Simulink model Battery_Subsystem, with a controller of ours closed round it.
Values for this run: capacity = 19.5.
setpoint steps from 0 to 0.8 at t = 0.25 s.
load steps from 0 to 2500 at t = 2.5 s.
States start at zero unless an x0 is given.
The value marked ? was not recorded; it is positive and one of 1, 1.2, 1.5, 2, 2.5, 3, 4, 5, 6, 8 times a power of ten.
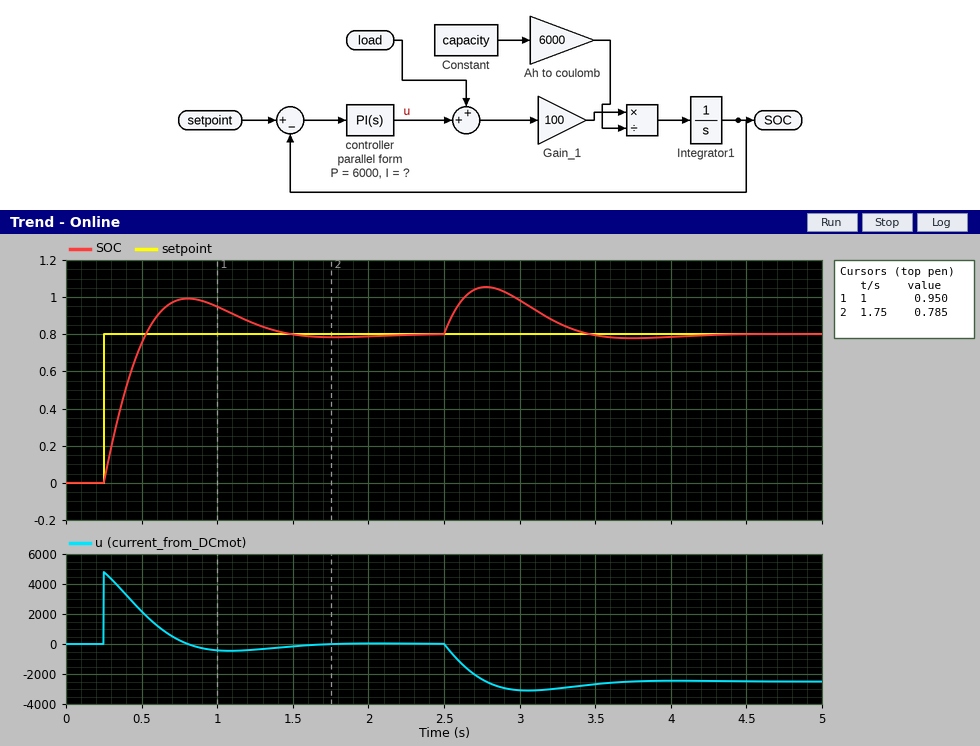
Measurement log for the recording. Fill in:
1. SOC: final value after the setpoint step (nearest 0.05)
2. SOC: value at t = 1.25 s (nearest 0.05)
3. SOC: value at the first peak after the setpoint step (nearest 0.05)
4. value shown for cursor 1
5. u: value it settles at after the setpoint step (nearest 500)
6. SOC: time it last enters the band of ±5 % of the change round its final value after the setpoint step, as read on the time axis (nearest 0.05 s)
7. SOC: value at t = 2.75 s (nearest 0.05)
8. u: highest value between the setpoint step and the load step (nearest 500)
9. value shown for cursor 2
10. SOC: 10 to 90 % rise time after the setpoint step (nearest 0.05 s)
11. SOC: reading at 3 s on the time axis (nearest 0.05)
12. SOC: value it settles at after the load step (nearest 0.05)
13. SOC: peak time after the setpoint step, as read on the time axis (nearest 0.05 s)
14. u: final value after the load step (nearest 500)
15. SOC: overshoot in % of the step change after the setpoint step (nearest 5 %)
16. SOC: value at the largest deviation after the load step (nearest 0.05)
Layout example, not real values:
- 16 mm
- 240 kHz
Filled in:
- 0.80
- 0.85
- 1.00
- 0.950
- 0
- 1.30 s
- 1.05
- 5000
- 0.785
- 0.20 s
- 1.00
- 0.80
- 0.80 s
- -2500
- 25 %
- 1.05
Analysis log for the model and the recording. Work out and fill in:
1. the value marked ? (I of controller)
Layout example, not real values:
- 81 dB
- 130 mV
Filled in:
- 20000
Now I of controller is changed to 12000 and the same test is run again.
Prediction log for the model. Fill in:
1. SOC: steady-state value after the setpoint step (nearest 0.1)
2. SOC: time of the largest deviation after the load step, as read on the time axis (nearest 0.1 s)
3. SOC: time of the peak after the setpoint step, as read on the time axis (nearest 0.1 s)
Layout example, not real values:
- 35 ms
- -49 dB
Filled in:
- 0.8
- 2.8 s
- 0.9 s
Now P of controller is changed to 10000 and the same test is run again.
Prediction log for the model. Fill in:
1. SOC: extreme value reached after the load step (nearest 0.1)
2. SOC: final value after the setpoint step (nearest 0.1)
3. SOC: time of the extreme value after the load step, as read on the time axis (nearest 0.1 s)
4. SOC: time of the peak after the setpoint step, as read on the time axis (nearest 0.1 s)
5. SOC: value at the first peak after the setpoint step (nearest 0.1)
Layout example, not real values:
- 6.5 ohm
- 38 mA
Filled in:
- 1.0
- 0.8
- 2.7 s
- 0.7 s
- 0.9
